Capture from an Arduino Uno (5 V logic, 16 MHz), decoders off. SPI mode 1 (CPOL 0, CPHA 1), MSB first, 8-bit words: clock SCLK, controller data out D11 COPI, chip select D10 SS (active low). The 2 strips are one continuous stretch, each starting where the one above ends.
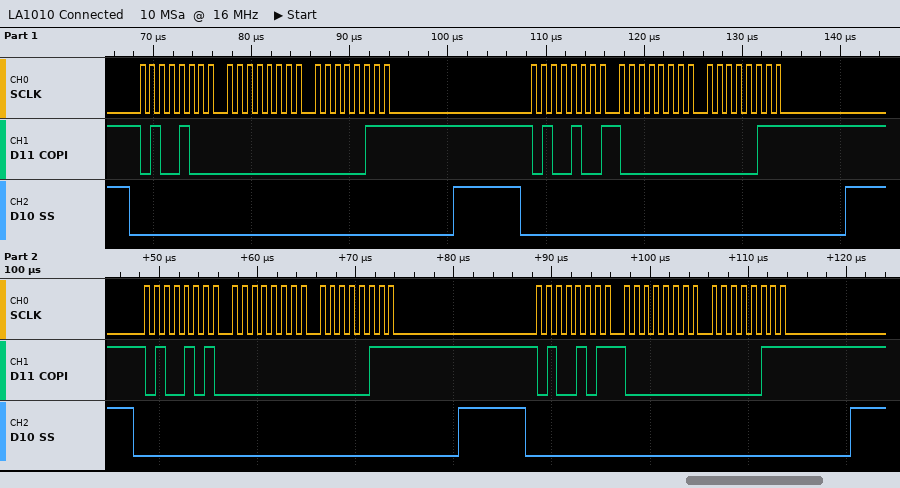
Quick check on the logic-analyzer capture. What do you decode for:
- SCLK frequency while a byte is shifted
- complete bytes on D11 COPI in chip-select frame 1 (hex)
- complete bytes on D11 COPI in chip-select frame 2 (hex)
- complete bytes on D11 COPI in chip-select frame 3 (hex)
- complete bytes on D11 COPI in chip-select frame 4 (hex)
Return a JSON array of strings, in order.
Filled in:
["1 MHz", "48 00 07", "49 00 07", "4A 00 07", "4B 00 07"]
